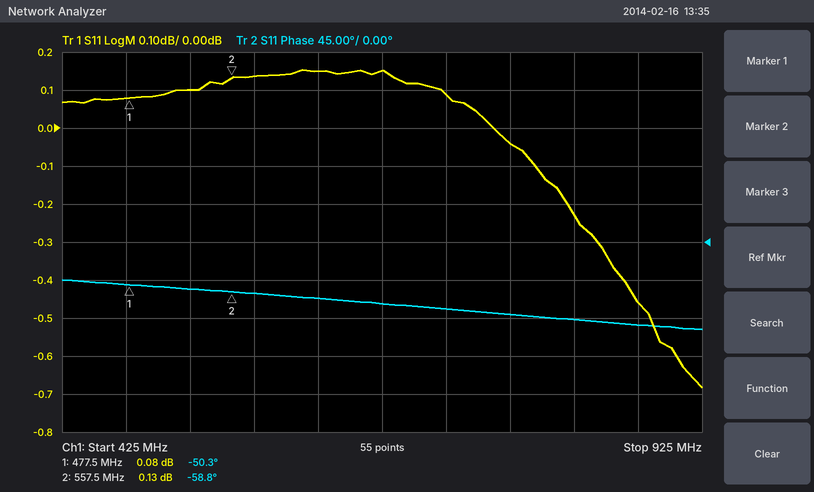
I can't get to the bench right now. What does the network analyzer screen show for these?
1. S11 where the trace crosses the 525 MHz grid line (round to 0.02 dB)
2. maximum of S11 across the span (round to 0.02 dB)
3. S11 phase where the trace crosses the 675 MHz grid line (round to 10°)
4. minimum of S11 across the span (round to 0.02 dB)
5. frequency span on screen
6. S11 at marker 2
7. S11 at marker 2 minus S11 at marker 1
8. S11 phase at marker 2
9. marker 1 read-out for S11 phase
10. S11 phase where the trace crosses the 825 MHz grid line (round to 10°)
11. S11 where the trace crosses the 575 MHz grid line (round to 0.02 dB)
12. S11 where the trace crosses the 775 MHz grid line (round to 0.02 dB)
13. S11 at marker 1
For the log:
0.10 dB
0.16 dB
-70°
-0.68 dB
500 MHz
0.13 dB
0.05 dB
-58.8°
-50.3°
-90°
0.14 dB
-0.04 dB
0.08 dB
